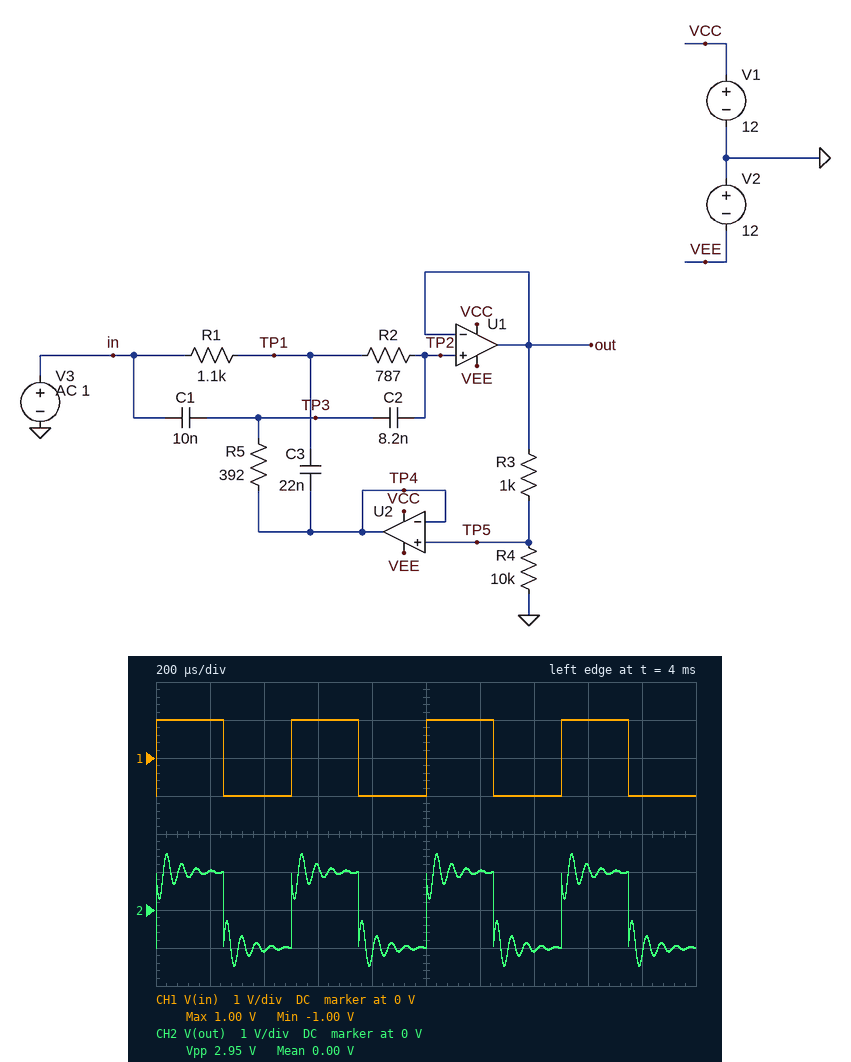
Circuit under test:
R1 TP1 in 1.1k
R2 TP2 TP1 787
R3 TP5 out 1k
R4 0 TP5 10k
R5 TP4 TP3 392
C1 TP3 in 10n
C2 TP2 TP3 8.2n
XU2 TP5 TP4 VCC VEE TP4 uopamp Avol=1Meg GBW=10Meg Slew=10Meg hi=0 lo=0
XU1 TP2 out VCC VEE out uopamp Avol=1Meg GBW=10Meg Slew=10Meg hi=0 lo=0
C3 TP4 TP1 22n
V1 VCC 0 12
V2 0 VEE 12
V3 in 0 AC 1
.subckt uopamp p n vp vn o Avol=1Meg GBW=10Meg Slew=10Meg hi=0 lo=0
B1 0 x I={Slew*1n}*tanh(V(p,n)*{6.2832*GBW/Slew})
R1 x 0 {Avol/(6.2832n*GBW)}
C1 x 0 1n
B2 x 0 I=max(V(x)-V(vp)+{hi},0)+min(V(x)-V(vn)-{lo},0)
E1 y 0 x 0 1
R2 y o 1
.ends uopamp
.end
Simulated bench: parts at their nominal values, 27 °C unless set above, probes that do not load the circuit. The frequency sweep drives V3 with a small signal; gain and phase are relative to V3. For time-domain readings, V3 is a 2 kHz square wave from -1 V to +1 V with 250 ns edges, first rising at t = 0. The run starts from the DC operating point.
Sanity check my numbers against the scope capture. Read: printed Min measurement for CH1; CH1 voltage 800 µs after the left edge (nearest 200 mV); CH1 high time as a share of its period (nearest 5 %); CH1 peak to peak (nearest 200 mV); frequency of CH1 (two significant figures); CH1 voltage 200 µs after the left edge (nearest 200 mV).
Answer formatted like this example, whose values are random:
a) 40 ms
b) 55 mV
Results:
a) -1.00 V
b) -1.0 V
c) 50 %
d) 2.0 V
e) 2.0 kHz
f) 1.0 V
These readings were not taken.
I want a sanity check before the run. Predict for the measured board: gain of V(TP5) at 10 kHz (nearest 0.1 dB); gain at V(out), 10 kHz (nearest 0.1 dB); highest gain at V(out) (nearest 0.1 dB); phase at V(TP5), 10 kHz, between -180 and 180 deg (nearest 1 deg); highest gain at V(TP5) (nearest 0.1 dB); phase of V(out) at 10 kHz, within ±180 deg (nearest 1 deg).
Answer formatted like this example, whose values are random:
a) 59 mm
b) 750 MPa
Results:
a) -0.9 dB
b) -0.1 dB
c) 0 dB
d) -18 deg
e) -0.8 dB
f) -18 deg
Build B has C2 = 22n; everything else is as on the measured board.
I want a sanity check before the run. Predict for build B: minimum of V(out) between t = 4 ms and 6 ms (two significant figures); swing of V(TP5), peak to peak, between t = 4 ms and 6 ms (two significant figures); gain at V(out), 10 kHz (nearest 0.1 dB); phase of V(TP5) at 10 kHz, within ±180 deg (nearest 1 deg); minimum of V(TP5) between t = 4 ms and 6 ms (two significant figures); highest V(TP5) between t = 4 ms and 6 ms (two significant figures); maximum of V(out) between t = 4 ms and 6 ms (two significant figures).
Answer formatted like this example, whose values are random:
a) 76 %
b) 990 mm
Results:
a) -1.2 V
b) 2.3 V
c) -3.2 dB
d) -36 deg
e) -1.1 V
f) 1.1 V
g) 1.2 V
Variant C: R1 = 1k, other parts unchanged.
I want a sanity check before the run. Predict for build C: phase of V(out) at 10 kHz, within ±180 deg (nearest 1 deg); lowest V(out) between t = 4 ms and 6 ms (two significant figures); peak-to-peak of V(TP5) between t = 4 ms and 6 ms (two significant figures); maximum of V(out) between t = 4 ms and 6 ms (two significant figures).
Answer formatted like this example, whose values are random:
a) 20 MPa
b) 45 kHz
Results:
a) -16 deg
b) -1.4 V
c) 2.6 V
d) 1.4 V
